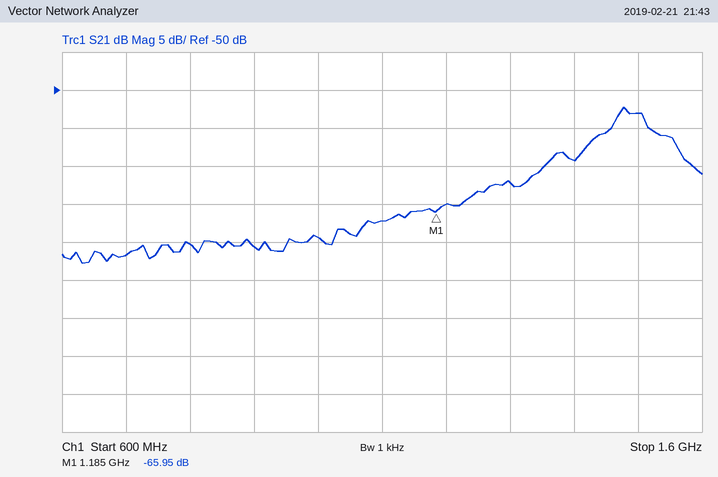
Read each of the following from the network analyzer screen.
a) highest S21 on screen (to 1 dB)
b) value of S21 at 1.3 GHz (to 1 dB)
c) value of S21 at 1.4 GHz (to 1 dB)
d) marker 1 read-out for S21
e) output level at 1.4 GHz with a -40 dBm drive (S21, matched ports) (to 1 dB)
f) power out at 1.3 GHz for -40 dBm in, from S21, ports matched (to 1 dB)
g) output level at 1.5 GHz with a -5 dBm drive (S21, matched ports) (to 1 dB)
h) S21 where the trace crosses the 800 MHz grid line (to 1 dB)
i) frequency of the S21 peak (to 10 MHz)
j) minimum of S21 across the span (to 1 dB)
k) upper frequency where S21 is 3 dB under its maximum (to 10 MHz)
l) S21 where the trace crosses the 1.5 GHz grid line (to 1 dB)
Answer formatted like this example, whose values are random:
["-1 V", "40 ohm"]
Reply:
["-52 dB", "-62 dB", "-59 dB", "-65.95 dB", "-99 dBm", "-102 dBm", "-58 dBm", "-70 dB", "1.48 GHz", "-73 dB", "1.52 GHz", "-53 dB"]
